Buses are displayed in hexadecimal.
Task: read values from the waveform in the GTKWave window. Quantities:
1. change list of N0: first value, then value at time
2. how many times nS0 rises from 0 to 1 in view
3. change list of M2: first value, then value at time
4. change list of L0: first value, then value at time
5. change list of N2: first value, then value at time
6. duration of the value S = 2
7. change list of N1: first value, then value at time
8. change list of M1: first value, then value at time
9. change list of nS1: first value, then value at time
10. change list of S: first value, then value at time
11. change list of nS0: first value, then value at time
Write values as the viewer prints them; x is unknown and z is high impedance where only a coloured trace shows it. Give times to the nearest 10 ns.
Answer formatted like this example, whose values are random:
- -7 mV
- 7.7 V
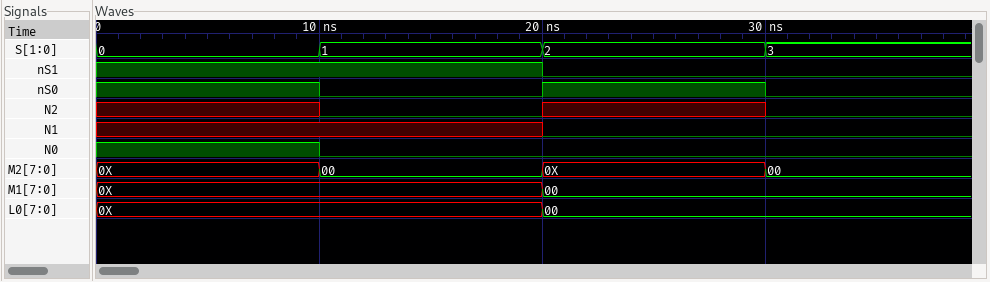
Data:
- 1, 0 at 10 ns
- 1
- 0X, 00 at 10 ns, 0X at 20 ns, 00 at 30 ns
- 0X, 00 at 20 ns
- x, 0 at 10 ns, x at 20 ns, 0 at 30 ns
- 10 ns
- x, 0 at 20 ns
- 0X, 00 at 20 ns
- 1, 0 at 20 ns
- 0, 1 at 10 ns, 2 at 20 ns, 3 at 30 ns
- 1, 0 at 10 ns, 1 at 20 ns, 0 at 30 ns
